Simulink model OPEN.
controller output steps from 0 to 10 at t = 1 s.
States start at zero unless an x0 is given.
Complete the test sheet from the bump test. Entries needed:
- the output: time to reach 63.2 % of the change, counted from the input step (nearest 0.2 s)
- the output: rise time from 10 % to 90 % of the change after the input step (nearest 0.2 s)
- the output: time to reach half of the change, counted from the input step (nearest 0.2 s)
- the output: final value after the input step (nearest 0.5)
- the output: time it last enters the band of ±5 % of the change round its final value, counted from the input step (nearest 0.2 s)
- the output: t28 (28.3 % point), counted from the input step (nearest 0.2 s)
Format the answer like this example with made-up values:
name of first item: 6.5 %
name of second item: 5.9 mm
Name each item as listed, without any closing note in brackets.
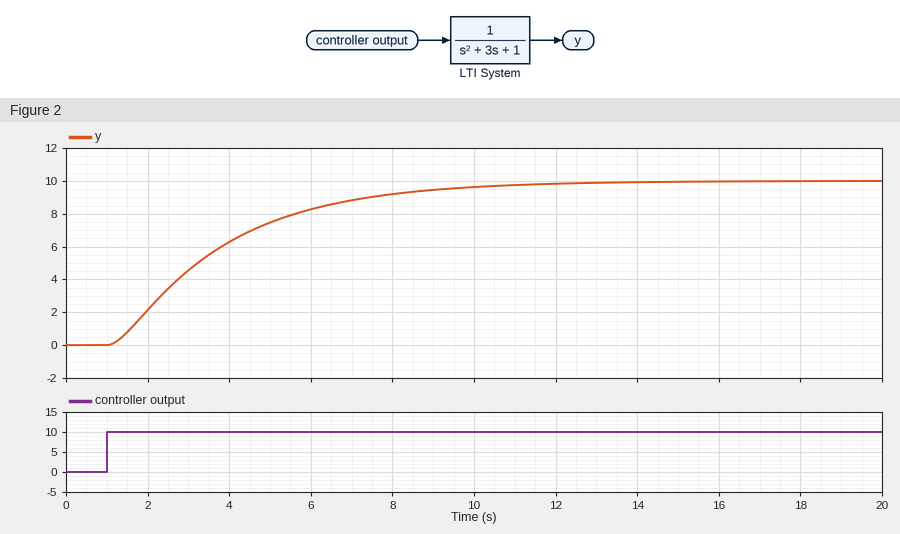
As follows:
the output: time to reach 63.2 % of the change, counted from the input step: 3.0 s
the output: rise time from 10 % to 90 % of the change after the input step: 5.8 s
the output: time to reach half of the change, counted from the input step: 2.2 s
the output: final value after the input step: 10.0
the output: time it last enters the band of ±5 % of the change round its final value, counted from the input step: 8.2 s
the output: t28 (28.3 % point), counted from the input step: 1.2 s
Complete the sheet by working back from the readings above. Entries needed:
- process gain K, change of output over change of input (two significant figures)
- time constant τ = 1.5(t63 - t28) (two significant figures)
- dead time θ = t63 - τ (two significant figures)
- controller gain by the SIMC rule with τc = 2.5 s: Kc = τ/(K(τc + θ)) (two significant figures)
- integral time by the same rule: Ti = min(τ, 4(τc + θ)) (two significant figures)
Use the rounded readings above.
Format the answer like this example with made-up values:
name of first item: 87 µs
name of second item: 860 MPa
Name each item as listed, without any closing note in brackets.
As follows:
process gain K, change of output over change of input: 1.0
time constant τ = 1.5(t63 - t28): 2.7 s
dead time θ = t63 - τ: 0.30 s
controller gain by the SIMC rule with τc = 2.5 s: Kc = τ/(K(τc + θ)): 0.96
integral time by the same rule: Ti = min(τ, 4(τc + θ)): 2.7 s
